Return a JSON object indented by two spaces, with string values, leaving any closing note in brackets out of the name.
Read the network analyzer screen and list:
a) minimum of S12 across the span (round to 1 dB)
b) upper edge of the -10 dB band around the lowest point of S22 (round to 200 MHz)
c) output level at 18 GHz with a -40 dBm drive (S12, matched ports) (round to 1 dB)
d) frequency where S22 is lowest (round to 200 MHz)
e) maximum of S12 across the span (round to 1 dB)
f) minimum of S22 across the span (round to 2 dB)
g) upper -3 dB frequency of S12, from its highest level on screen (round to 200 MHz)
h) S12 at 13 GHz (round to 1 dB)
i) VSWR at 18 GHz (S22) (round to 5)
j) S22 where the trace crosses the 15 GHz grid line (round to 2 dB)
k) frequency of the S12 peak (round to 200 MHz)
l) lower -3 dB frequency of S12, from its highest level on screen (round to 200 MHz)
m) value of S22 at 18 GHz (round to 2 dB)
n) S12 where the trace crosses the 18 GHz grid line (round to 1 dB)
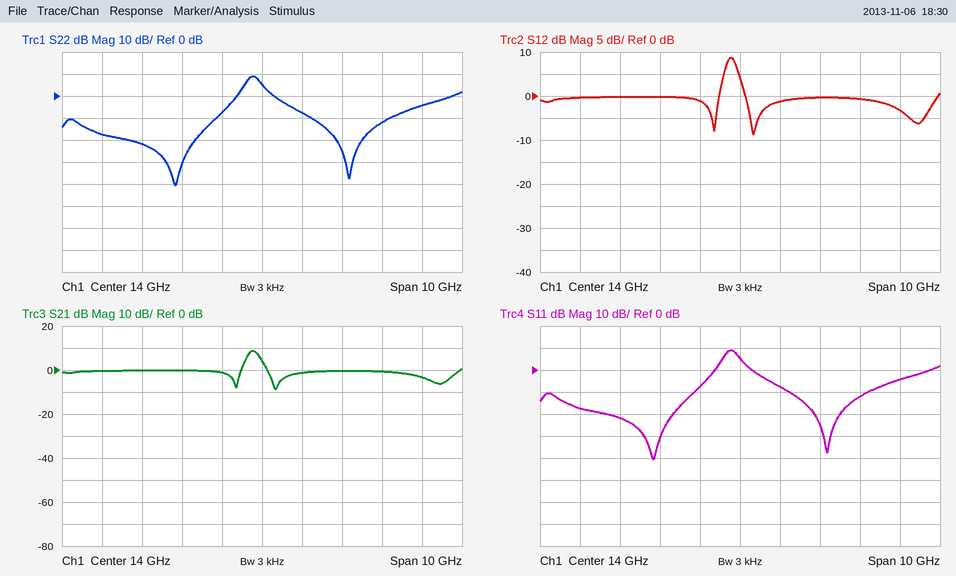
{
  "minimum of S12 across the span": "-9 dB",
  "upper edge of the -10 dB band around the lowest point of S22": "12.8 GHz",
  "output level at 18 GHz with a -40 dBm drive (S12, matched ports)": "-43 dBm",
  "frequency where S22 is lowest": "11.8 GHz",
  "maximum of S12 across the span": "9 dB",
  "minimum of S22 across the span": "-40 dB",
  "upper -3 dB frequency of S12, from its highest level on screen": "14.0 GHz",
  "S12 at 13 GHz": "-1 dB",
  "VSWR at 18 GHz (S22)": "5",
  "S22 where the trace crosses the 15 GHz grid line": "-8 dB",
  "frequency of the S12 peak": "13.8 GHz",
  "lower -3 dB frequency of S12, from its highest level on screen": "13.6 GHz",
  "value of S22 at 18 GHz": "-4 dB",
  "S12 where the trace crosses the 18 GHz grid line": "-3 dB"
}
